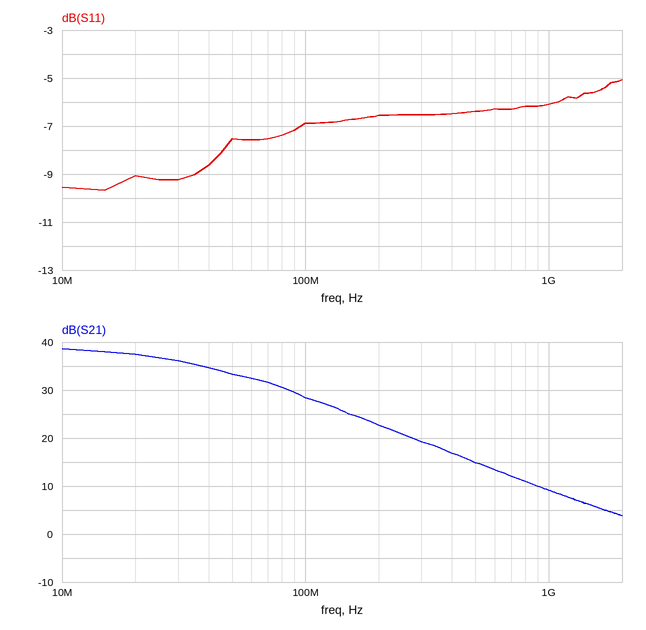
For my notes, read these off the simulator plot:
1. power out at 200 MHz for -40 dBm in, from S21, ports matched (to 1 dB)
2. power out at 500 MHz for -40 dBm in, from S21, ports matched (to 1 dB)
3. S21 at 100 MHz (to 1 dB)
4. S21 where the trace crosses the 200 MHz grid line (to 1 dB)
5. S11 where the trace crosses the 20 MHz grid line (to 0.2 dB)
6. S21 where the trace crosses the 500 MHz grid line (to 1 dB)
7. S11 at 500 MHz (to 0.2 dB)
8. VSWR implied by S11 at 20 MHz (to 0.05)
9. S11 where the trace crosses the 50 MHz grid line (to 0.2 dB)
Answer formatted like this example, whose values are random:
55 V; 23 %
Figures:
-17 dBm; -25 dBm; 28 dB; 23 dB; -9.0 dB; 15 dB; -6.4 dB; 2.10; -7.6 dB
